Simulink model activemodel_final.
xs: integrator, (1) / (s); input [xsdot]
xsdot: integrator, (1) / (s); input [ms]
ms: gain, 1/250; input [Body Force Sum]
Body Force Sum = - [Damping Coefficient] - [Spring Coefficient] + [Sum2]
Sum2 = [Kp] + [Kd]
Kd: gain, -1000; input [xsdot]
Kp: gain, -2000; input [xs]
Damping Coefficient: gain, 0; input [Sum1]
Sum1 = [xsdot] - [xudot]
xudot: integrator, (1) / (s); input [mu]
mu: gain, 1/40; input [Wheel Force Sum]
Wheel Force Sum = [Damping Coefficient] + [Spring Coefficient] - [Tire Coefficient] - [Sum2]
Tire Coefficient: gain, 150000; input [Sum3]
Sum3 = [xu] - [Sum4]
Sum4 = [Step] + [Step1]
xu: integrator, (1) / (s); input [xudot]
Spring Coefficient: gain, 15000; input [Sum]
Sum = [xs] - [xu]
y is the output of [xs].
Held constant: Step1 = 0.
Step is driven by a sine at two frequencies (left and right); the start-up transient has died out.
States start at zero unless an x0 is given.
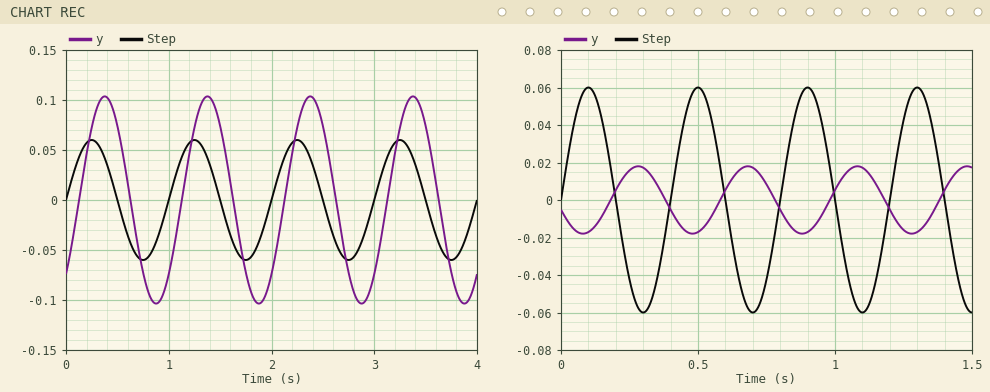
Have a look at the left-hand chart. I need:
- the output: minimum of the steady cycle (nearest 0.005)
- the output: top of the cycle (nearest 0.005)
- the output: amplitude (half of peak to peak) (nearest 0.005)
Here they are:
-0.105
0.105
0.105
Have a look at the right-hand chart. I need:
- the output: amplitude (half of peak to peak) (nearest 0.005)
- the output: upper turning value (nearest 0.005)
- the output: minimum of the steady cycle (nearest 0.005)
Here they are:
0.020
0.020
-0.020
